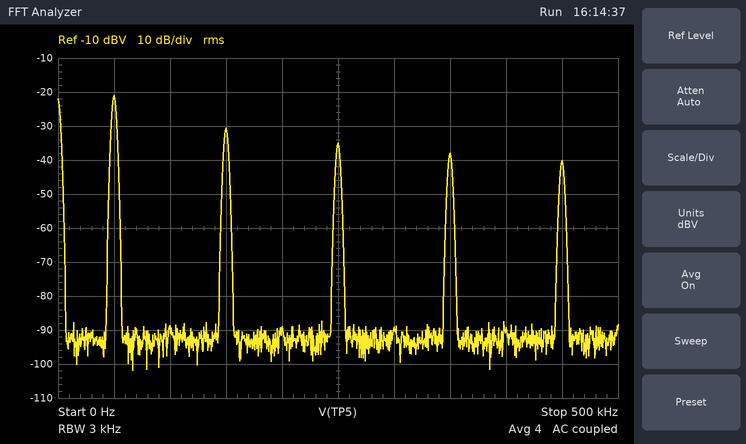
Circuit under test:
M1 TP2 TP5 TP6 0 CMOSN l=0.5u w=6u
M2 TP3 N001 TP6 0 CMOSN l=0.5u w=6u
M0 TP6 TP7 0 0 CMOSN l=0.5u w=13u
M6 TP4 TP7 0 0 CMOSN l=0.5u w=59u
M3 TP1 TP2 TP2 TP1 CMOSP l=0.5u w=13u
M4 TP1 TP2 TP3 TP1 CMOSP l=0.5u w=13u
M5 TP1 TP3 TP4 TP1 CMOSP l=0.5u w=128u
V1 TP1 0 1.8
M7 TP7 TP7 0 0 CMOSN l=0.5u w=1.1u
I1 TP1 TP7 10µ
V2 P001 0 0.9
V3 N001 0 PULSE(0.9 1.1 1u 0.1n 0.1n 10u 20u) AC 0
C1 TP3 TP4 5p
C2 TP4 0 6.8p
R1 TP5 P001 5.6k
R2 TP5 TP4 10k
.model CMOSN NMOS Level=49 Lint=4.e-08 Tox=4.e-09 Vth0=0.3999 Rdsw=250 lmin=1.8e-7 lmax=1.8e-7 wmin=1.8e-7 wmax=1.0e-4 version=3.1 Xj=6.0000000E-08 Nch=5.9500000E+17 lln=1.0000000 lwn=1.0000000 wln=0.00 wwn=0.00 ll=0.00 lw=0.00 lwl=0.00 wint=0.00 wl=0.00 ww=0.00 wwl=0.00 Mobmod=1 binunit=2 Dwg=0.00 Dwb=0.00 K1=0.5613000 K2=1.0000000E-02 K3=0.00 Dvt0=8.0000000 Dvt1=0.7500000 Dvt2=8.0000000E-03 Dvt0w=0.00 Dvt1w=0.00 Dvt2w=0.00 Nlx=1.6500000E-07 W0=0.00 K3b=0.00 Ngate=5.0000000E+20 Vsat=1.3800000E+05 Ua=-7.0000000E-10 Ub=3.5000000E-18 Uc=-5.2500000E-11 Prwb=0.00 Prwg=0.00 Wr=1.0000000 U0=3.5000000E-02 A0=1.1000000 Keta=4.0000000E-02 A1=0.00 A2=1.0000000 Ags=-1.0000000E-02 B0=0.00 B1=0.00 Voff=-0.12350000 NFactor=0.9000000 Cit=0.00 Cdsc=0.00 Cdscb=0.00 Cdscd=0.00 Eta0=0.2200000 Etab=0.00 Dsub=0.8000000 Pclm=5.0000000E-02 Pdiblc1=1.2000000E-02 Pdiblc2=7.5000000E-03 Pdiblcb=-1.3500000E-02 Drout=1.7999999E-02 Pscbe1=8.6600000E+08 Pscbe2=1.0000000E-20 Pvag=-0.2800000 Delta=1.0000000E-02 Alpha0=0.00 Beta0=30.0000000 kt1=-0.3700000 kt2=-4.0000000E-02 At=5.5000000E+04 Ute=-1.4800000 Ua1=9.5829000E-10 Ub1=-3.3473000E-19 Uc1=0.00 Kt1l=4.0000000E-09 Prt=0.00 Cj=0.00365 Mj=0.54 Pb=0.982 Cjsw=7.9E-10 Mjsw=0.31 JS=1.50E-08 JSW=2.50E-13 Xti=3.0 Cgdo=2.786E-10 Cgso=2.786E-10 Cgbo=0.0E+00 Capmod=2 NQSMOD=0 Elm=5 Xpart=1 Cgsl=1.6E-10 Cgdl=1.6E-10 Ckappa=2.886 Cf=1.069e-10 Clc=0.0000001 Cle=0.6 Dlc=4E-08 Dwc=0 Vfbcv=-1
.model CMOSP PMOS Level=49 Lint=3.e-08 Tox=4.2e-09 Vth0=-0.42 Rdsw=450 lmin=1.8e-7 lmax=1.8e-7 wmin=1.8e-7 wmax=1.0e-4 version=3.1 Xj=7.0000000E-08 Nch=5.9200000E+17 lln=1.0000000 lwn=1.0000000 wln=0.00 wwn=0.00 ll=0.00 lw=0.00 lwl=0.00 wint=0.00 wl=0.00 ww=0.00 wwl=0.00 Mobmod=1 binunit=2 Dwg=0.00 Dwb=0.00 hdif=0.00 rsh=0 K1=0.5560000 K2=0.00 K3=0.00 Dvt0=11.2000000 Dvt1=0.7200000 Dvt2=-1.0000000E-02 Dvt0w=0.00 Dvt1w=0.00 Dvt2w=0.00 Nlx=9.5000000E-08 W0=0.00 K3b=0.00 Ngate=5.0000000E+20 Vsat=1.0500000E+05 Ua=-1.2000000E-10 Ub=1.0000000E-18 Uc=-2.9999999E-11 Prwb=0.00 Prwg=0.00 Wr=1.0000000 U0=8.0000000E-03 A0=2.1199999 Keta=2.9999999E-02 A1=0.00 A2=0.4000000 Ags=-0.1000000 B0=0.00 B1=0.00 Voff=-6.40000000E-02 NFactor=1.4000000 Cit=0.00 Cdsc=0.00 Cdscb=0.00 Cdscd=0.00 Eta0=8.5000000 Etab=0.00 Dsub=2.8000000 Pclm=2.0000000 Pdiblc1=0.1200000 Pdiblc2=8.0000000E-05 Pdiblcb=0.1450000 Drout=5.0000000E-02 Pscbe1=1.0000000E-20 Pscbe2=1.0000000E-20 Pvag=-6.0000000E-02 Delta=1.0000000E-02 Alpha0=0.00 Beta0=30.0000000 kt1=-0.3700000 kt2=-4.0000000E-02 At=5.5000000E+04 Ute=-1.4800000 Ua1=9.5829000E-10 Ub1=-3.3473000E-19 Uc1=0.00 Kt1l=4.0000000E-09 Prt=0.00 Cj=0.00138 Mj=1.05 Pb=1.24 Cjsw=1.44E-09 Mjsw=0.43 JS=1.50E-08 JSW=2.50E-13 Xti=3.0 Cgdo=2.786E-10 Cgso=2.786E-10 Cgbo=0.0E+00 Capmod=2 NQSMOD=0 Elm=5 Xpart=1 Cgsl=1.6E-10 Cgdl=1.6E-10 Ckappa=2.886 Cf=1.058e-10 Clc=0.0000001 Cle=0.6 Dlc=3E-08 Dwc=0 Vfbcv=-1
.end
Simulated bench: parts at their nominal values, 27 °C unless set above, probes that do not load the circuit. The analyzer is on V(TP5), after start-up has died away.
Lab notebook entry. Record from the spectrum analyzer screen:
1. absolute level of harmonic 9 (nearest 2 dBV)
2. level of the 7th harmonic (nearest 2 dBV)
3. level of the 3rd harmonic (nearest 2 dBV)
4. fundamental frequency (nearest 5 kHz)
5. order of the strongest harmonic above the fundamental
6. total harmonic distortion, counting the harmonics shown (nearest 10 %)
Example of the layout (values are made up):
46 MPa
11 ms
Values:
-40 dBV
-38 dBV
-30 dBV
50 kHz
3
40 %
